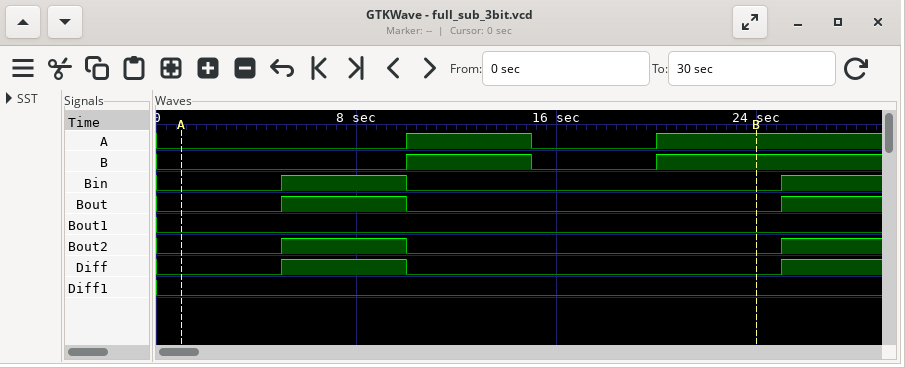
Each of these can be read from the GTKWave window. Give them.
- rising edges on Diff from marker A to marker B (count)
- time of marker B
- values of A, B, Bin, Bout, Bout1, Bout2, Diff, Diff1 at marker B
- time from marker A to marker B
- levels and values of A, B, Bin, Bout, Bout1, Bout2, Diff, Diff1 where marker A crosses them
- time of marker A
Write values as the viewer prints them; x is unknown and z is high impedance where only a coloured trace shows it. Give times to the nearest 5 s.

1
25 s
A=1, B=1, Bin=0, Bout=0, Bout1=0, Bout2=0, Diff=0, Diff1=0
25 s
A=0, B=0, Bin=0, Bout=0, Bout1=0, Bout2=0, Diff=0, Diff1=0
0 s
